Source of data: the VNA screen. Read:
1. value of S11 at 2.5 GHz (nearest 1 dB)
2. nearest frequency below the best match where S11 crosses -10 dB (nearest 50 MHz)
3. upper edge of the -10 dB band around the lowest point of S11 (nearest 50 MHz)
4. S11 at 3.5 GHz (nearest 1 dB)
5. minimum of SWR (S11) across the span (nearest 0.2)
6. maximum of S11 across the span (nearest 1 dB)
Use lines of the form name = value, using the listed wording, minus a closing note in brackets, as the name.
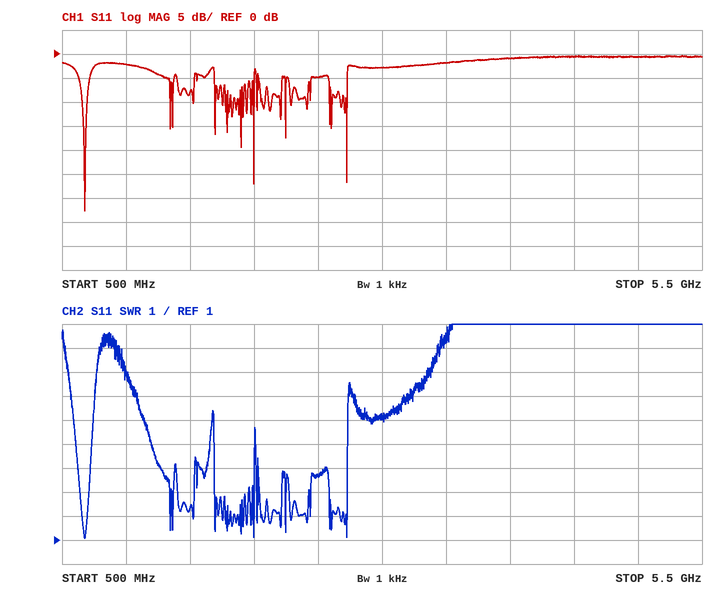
value of S11 at 2.5 GHz = -5 dB
nearest frequency below the best match where S11 crosses -10 dB = 650 MHz
upper edge of the -10 dB band around the lowest point of S11 = 700 MHz
S11 at 3.5 GHz = -2 dB
minimum of SWR (S11) across the span = 1.0
maximum of S11 across the span = 0 dB
